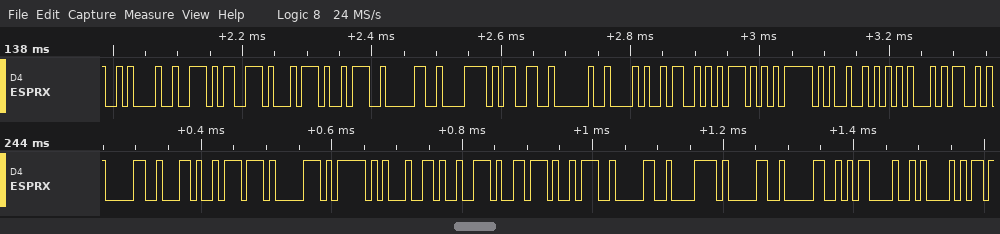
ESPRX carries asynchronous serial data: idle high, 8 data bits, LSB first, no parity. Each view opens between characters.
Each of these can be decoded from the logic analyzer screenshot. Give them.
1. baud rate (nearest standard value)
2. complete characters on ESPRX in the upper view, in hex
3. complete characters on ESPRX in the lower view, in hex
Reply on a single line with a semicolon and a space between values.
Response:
115200 baud; 0A, 72, 73, 74, 3A, 30, 78, 33, 20, 28, 53, 57, 5F, 52, 45; 30, 2C, 77, 70, 5F, 64, 72, 76, 3A, 30, 78, 30, 30, 0D, 0A
